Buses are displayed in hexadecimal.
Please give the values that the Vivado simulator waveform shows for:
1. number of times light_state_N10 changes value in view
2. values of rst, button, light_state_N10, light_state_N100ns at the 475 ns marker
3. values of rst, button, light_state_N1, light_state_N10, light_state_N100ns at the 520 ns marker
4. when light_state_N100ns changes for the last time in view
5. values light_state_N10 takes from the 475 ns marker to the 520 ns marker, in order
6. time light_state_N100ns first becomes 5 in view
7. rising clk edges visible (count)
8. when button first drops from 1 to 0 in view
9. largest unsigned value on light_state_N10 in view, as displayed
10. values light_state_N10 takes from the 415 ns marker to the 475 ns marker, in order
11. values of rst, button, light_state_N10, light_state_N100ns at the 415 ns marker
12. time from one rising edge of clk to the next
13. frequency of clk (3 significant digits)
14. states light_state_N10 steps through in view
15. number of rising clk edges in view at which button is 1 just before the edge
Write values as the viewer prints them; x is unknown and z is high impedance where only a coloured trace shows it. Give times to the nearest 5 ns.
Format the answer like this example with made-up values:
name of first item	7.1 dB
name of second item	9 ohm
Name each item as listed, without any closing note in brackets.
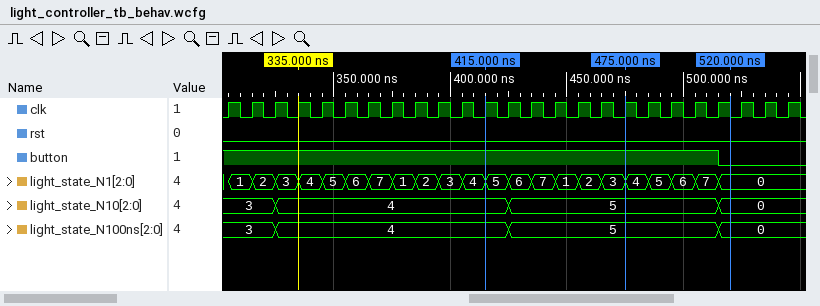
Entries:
number of times light_state_N10 changes value in view	3
values of rst, button, light_state_N10, light_state_N100ns at the 475 ns marker	rst=0, button=1, light_state_N10=5, light_state_N100ns=5
values of rst, button, light_state_N1, light_state_N10, light_state_N100ns at the 520 ns marker	rst=0, button=0, light_state_N1=0, light_state_N10=0, light_state_N100ns=0
when light_state_N100ns changes for the last time in view	515 ns
values light_state_N10 takes from the 475 ns marker to the 520 ns marker, in order	5, 0
time light_state_N100ns first becomes 5 in view	425 ns
rising clk edges visible	25
when button first drops from 1 to 0 in view	515 ns
largest unsigned value on light_state_N10 in view, as displayed	5
values light_state_N10 takes from the 415 ns marker to the 475 ns marker, in order	4, 5
values of rst, button, light_state_N10, light_state_N100ns at the 415 ns marker	rst=0, button=1, light_state_N10=4, light_state_N100ns=4
time from one rising edge of clk to the next	10 ns
frequency of clk	100 MHz
states light_state_N10 steps through in view	3, 4, 5, 0
number of rising clk edges in view at which button is 1 just before the edge	22
